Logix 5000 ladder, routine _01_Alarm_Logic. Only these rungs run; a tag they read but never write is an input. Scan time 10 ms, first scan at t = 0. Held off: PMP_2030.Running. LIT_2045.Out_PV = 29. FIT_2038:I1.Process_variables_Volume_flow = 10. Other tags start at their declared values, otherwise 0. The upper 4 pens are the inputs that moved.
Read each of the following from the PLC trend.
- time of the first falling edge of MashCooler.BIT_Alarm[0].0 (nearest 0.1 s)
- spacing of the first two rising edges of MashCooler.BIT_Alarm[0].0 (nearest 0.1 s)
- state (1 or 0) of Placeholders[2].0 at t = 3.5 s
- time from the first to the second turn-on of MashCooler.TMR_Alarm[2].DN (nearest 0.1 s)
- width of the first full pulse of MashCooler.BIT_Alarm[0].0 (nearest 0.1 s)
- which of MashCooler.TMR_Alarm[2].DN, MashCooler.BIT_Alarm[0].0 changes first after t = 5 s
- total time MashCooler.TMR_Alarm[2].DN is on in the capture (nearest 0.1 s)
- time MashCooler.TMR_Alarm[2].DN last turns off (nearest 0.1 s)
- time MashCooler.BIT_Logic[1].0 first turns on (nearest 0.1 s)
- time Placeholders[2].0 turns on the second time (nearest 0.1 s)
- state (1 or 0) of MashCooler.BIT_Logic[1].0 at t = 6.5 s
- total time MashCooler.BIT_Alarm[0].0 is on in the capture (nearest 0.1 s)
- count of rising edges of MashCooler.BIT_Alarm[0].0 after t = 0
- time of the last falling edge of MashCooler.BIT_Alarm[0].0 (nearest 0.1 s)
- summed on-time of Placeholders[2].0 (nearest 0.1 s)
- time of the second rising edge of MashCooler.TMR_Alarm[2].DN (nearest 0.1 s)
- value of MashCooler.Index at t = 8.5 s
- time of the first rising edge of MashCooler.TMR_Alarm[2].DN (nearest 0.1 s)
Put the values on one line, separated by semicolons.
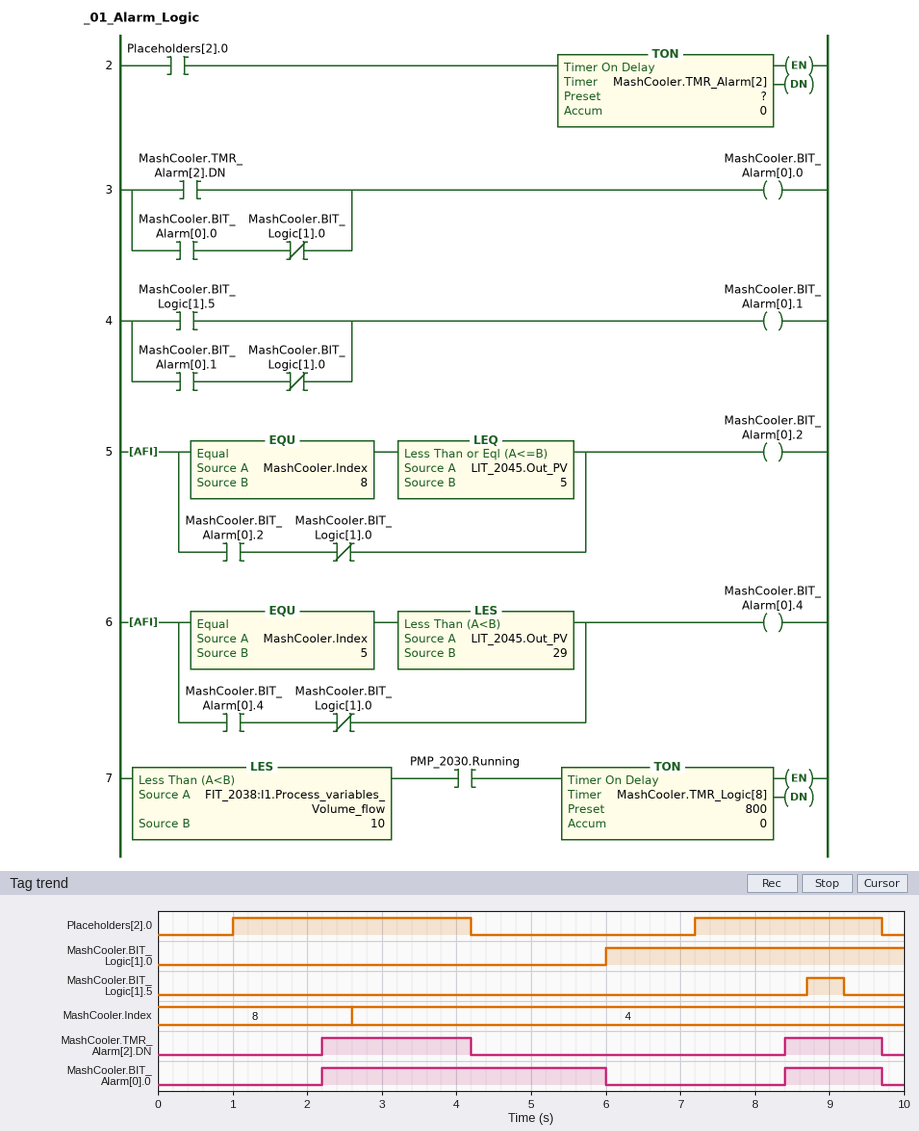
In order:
6.0 s; 6.2 s; 1; 6.2 s; 3.8 s; MashCooler.BIT_Alarm[0].0; 3.3 s; 9.7 s; 6.0 s; 7.2 s; 1; 5.1 s; 2; 9.7 s; 5.7 s; 8.4 s; 4; 2.2 s
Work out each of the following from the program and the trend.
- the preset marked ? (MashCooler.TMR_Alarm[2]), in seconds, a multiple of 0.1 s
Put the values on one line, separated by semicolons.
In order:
1.2 s
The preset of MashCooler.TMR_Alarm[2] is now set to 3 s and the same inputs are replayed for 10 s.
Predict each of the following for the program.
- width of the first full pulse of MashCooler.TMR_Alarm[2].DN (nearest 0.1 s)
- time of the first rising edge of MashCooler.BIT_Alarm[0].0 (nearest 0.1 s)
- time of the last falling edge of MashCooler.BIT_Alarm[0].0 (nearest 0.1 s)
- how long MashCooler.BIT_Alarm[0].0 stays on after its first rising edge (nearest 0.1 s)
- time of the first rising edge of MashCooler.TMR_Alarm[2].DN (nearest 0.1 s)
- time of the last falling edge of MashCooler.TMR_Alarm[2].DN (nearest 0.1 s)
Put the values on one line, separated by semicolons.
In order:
0.2 s; 4.0 s; 6.0 s; 2.0 s; 4.0 s; 4.2 s
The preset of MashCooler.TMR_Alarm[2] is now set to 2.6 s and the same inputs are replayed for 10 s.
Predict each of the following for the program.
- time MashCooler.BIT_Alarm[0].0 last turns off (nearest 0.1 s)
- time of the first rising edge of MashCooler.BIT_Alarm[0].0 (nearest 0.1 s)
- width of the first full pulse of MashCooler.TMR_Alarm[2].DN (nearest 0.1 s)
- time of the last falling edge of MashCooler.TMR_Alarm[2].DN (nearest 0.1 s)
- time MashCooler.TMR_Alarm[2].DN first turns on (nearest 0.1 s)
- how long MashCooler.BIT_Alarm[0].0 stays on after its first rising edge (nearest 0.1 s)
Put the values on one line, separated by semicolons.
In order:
6.0 s; 3.6 s; 0.6 s; 4.2 s; 3.6 s; 2.4 s
